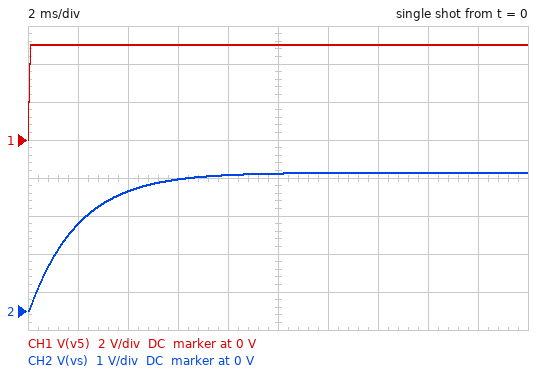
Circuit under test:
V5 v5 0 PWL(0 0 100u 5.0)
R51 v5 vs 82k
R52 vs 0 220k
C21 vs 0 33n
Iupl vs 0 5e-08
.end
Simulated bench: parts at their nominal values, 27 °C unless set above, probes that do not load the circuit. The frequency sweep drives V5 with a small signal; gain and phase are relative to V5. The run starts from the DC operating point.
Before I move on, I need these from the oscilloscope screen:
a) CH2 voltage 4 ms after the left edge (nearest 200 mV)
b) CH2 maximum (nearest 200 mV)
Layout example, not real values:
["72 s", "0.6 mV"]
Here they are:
["3.2 V", "3.6 V"]
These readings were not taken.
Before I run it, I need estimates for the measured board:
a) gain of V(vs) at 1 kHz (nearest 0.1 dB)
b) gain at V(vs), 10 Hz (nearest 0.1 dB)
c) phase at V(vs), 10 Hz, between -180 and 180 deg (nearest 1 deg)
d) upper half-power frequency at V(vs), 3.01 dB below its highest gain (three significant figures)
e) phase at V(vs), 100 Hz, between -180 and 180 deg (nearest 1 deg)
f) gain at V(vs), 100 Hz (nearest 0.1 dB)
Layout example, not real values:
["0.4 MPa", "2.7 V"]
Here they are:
["-24.6 dB", "-2.8 dB", "-7 deg", "80.7 Hz", "-51 deg", "-6.8 dB"]
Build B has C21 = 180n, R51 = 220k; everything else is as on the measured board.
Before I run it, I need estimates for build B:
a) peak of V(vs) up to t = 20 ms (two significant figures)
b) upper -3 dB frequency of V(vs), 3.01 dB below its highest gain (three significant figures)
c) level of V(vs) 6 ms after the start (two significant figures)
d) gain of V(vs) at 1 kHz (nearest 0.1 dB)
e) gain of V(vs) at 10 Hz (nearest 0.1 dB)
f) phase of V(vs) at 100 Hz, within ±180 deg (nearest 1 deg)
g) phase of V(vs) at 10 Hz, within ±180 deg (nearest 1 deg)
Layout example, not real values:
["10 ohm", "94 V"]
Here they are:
["1.6 V", "8.04 Hz", "640 mV", "-47.9 dB", "-10.1 dB", "-85 deg", "-51 deg"]
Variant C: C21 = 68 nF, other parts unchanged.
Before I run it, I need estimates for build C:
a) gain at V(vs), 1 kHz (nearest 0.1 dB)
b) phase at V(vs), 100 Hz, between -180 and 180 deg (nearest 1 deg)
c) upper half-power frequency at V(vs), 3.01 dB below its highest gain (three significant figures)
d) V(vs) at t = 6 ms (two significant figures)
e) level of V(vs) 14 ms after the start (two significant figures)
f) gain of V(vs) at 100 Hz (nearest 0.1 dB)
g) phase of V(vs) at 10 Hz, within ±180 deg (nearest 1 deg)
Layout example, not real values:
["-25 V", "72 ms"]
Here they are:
["-30.9 dB", "-69 deg", "39.2 Hz", "2.8 V", "3.5 V", "-11.5 dB", "-14 deg"]
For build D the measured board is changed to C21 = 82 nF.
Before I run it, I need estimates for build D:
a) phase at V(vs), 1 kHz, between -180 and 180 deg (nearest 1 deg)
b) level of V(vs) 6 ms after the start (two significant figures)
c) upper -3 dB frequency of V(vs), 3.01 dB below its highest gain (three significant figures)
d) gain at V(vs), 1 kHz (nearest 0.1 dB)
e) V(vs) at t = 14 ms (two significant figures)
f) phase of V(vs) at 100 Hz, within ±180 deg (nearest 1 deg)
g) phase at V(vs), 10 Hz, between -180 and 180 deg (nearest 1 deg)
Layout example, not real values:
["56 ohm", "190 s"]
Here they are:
["-88 deg", "2.6 V", "32.5 Hz", "-32.5 dB", "3.4 V", "-72 deg", "-17 deg"]
